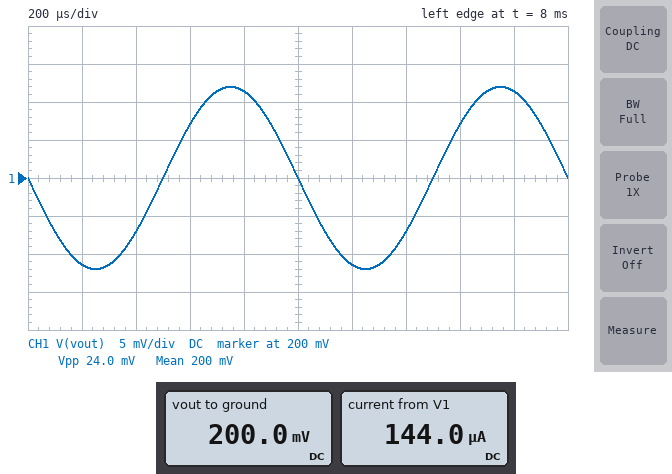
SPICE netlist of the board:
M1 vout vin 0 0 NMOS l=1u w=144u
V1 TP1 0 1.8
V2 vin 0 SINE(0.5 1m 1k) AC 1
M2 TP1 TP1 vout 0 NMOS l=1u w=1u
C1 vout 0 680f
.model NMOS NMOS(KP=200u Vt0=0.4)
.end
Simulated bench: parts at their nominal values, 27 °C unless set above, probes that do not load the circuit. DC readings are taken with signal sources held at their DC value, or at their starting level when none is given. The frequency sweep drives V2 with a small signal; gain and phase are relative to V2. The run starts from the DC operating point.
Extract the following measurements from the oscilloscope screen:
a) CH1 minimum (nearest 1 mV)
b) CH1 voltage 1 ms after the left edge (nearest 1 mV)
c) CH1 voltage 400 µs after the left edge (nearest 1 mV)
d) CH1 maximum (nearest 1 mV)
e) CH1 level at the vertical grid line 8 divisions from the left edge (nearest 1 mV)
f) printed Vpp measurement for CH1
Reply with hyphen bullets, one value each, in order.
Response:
- 188 mV
- 200 mV
- 193 mV
- 212 mV
- 207 mV
- 24.0 mV
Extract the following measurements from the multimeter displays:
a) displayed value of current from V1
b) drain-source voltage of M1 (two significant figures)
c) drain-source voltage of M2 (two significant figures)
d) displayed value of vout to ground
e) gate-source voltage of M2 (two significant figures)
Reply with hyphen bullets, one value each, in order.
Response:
- 144.0 µA
- 200 mV
- 1.6 V
- 200.0 mV
- 1.6 V
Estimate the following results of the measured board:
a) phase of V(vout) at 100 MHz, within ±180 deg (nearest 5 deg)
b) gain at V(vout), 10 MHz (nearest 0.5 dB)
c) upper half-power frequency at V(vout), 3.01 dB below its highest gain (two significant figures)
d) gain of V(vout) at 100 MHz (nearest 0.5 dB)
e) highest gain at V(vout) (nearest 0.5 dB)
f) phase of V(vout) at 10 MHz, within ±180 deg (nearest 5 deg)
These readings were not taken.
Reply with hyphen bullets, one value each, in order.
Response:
- 120 deg
- 21.5 dB
- 56 MHz
- 15.5 dB
- 21.5 dB
- 170 deg
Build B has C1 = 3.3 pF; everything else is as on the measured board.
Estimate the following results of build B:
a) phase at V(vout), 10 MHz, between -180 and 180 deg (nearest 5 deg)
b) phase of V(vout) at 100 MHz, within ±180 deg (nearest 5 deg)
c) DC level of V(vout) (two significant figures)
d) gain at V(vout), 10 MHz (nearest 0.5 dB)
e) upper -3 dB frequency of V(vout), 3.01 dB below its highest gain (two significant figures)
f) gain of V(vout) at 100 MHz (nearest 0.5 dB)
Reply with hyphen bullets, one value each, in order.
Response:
- 140 deg
- 95 deg
- 200 mV
- 19.0 dB
- 12 MHz
- 3.0 dB
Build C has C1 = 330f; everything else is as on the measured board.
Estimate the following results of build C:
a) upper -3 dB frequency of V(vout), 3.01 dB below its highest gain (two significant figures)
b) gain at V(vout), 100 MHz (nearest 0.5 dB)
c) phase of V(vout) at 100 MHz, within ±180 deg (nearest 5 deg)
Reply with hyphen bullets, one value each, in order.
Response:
- 120 MHz
- 19.0 dB
- 140 deg
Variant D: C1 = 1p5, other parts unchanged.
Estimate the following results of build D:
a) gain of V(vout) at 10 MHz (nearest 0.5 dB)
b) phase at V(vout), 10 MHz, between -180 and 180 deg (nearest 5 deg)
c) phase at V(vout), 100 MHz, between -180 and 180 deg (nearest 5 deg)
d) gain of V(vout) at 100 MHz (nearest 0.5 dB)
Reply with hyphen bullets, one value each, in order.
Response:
- 21.0 dB
- 160 deg
- 105 deg
- 9.5 dB
